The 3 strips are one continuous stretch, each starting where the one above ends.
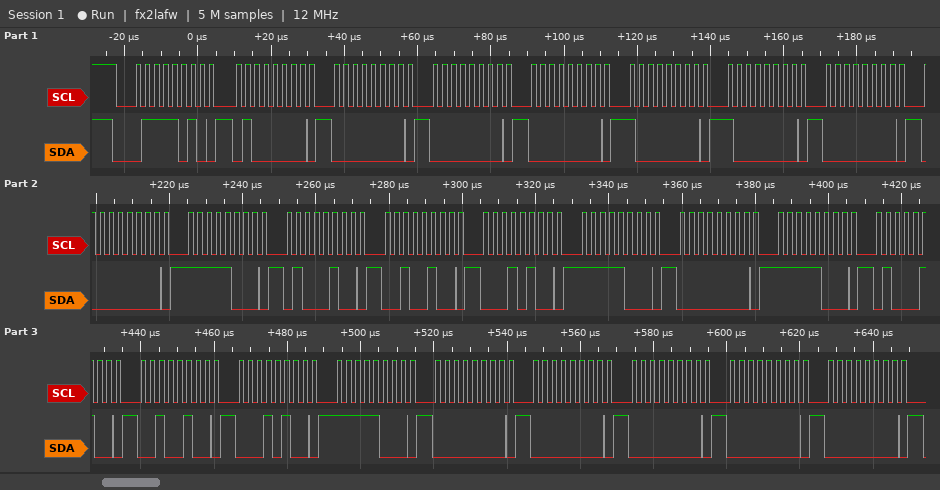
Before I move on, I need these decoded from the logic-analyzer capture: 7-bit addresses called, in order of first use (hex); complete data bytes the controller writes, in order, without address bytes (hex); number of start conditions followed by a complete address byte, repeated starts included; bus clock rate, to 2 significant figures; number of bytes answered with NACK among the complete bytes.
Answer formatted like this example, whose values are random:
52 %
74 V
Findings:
0x3D
40 00 00 00 80 80 00 00 F8 44 24 14 F8 00 F8 44 24 14 F8 00 00 00 00 00
1
400 kHz
0
